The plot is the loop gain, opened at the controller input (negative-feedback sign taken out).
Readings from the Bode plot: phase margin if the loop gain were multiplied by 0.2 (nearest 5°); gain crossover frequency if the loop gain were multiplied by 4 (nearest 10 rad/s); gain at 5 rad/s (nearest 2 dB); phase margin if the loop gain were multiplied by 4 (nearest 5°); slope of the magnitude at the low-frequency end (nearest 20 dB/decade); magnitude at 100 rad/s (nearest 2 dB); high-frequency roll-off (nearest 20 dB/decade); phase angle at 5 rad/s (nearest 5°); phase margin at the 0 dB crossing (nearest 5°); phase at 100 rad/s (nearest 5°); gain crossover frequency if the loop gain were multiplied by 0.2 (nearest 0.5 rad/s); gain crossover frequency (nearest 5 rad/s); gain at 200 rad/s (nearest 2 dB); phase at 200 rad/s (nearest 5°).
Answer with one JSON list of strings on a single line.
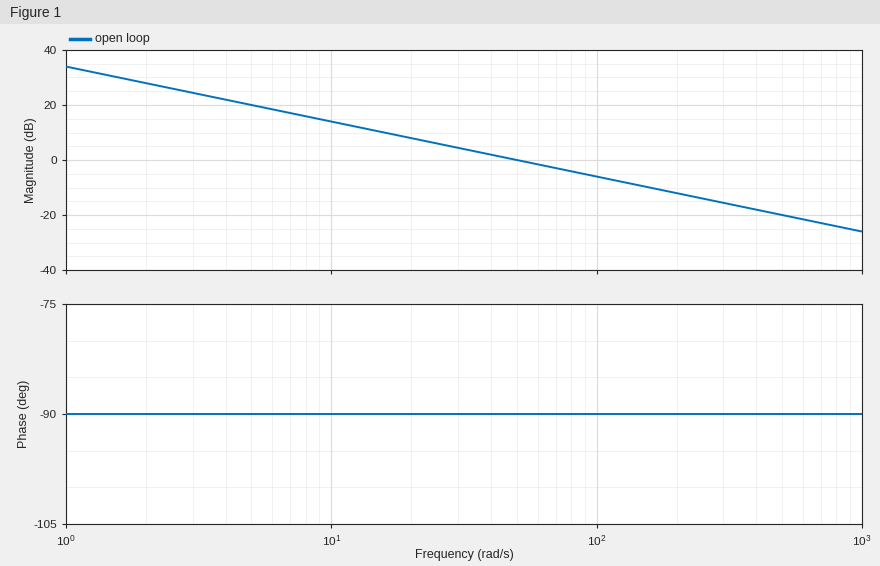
["90°", "200 rad/s", "20 dB", "90°", "-20 dB/decade", "-6 dB", "-20 dB/decade", "-90°", "90°", "-90°", "10.0 rad/s", "50 rad/s", "-12 dB", "-90°"]
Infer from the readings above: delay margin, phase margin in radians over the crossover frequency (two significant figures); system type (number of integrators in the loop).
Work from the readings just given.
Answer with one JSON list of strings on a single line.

["0.031 s", "1"]
